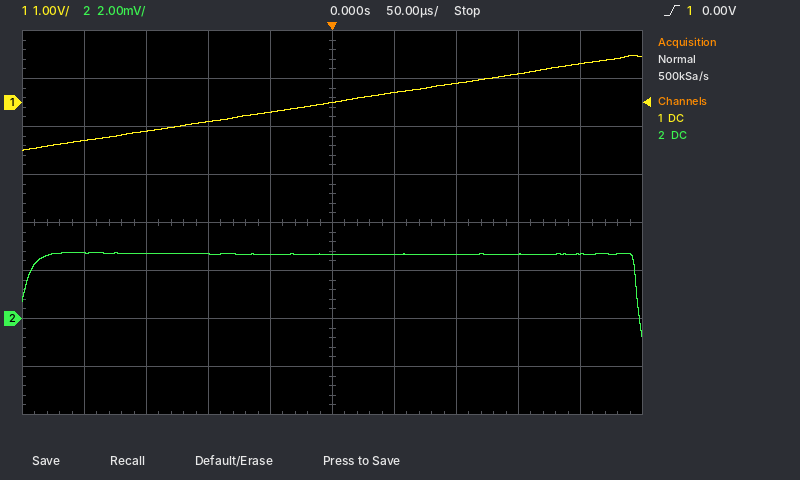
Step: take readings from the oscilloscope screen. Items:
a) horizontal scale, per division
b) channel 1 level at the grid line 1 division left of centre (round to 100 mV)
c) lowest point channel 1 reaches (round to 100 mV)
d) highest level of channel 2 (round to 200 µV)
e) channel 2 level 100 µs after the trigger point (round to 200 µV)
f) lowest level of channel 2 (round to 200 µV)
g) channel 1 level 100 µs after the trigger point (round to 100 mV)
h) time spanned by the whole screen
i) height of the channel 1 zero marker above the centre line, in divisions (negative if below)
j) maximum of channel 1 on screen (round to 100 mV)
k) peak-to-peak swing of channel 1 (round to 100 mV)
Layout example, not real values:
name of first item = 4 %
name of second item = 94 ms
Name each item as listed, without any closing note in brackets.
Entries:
horizontal scale, per division = 50 µs
channel 1 level at the grid line 1 division left of centre = -200 mV
lowest point channel 1 reaches = -1.0 V
highest level of channel 2 = 2.8 mV
channel 2 level 100 µs after the trigger point = 2.6 mV
lowest level of channel 2 = -800 µV
channel 1 level 100 µs after the trigger point = 400 mV
time spanned by the whole screen = 500 µs
height of the channel 1 zero marker above the centre line, in divisions = +2.5 div
maximum of channel 1 on screen = 1.0 V
peak-to-peak swing of channel 1 = 2.0 V
